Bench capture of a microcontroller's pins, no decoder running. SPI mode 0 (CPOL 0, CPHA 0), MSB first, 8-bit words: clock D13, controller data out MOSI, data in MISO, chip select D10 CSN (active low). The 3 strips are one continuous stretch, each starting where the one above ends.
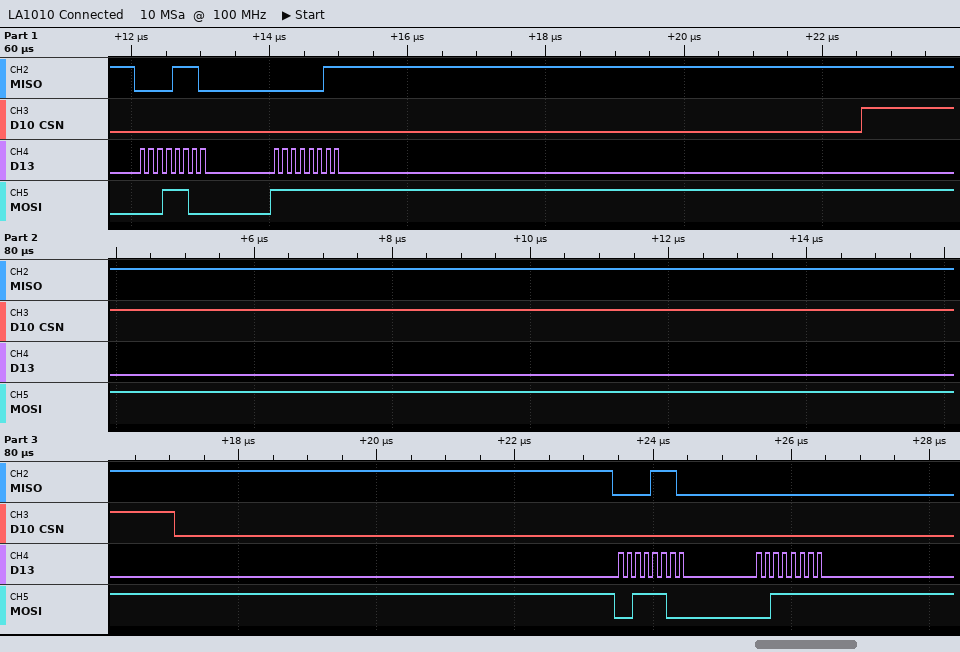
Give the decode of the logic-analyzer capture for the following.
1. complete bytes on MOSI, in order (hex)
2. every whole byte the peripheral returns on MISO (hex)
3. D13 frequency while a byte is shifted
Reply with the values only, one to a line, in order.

1C FF 3C 3F
0E 03 0E 00
8 MHz
